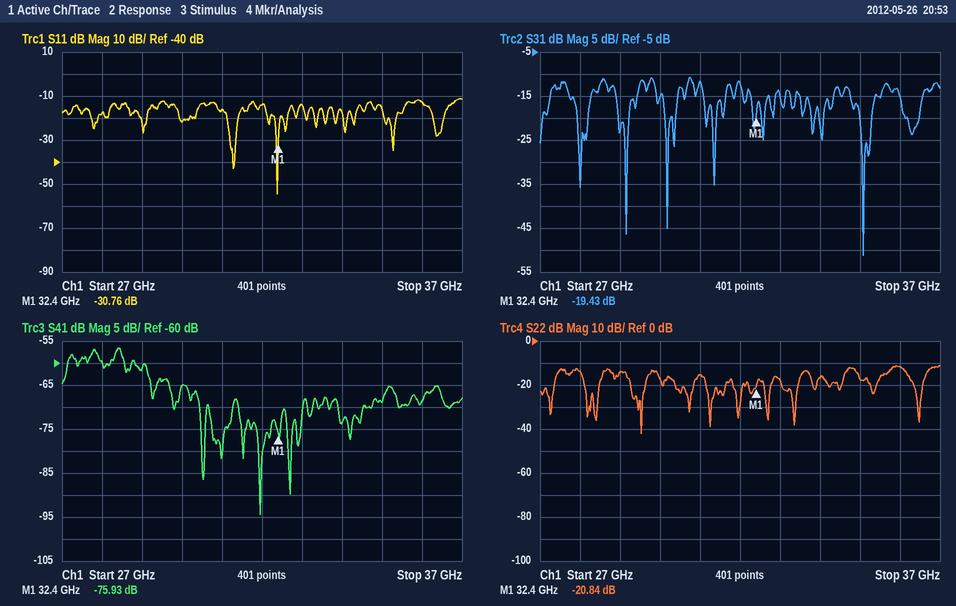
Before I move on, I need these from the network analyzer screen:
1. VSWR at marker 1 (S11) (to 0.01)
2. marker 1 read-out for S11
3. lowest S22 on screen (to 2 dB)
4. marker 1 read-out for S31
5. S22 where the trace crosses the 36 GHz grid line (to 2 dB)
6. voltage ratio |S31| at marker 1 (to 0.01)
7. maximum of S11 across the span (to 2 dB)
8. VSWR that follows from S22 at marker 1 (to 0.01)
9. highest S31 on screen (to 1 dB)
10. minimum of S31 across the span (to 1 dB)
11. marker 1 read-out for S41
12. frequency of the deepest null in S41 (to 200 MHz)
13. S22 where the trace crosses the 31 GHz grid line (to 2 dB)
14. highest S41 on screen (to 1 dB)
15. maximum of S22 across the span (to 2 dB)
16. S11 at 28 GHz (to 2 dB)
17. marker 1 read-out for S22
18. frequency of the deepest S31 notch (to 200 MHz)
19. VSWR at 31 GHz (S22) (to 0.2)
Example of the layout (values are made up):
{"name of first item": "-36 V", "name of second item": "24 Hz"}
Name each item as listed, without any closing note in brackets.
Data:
{"VSWR at marker 1 (S11)": "1.06", "marker 1 read-out for S11": "-30.76 dB", "lowest S22 on screen": "-42 dB", "marker 1 read-out for S31": "-19.43 dB", "S22 where the trace crosses the 36 GHz grid line": "-12 dB", "voltage ratio |S31| at marker 1": "0.11", "maximum of S11 across the span": "-12 dB", "VSWR that follows from S22 at marker 1": "1.20", "highest S31 on screen": "-11 dB", "minimum of S31 across the span": "-51 dB", "marker 1 read-out for S41": "-75.93 dB", "frequency of the deepest null in S41": "32.0 GHz", "S22 where the trace crosses the 31 GHz grid line": "-16 dB", "highest S41 on screen": "-57 dB", "maximum of S22 across the span": "-12 dB", "S11 at 28 GHz": "-18 dB", "marker 1 read-out for S22": "-20.84 dB", "frequency of the deepest S31 notch": "35.0 GHz", "VSWR at 31 GHz (S22)": "1.4"}
